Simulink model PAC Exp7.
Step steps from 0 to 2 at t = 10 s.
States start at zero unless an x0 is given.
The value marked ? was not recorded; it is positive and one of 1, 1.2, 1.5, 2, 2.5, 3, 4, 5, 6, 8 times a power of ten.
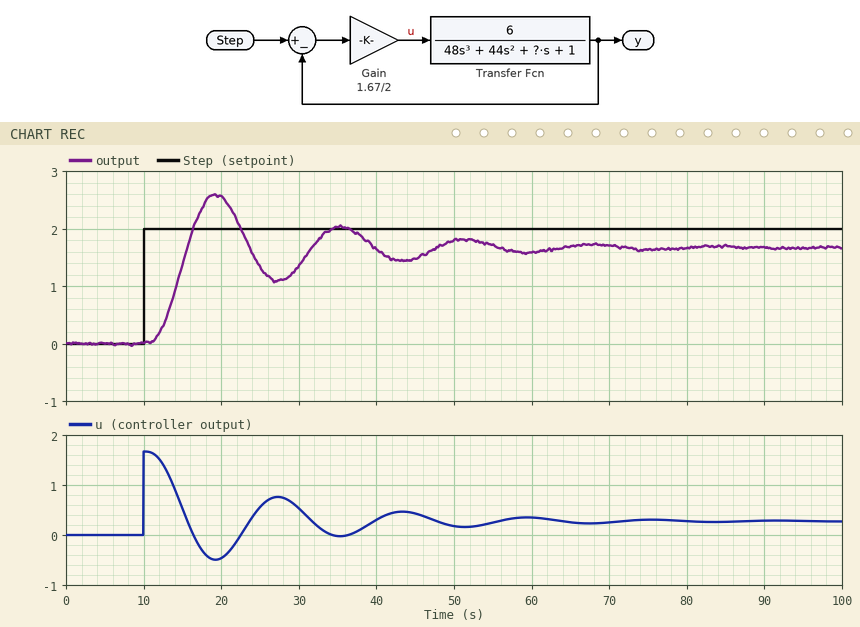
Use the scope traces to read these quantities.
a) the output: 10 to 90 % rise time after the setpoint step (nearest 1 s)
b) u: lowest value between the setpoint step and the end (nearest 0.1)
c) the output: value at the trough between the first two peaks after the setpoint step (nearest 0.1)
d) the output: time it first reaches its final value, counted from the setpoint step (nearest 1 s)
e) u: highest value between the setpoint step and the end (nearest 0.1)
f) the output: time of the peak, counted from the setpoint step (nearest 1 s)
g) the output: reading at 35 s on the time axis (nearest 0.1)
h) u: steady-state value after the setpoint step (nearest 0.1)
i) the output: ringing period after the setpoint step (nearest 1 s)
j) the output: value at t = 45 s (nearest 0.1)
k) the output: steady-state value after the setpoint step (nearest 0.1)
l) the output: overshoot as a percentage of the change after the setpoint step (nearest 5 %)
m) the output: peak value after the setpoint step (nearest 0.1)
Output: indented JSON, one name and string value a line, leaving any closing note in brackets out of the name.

{
  "the output: 10 to 90 % rise time after the setpoint step": "3 s",
  "u: lowest value between the setpoint step and the end": "-0.5",
  "the output: value at the trough between the first two peaks after the setpoint step": "1.1",
  "the output: time it first reaches its final value, counted from the setpoint step": "6 s",
  "u: highest value between the setpoint step and the end": "1.7",
  "the output: time of the peak, counted from the setpoint step": "9 s",
  "the output: reading at 35 s on the time axis": "2.0",
  "u: steady-state value after the setpoint step": "0.3",
  "the output: ringing period after the setpoint step": "16 s",
  "the output: value at t = 45 s": "1.5",
  "the output: steady-state value after the setpoint step": "1.7",
  "the output: overshoot as a percentage of the change after the setpoint step": "55 %",
  "the output: peak value after the setpoint step": "2.6"
}
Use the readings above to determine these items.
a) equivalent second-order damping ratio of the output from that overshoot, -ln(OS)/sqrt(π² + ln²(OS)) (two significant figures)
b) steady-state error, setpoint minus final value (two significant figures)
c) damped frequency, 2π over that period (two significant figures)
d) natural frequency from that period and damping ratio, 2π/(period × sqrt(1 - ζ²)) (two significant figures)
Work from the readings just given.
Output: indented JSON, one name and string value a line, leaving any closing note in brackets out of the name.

{
  "equivalent second-order damping ratio of the output from that overshoot, -ln(OS)/sqrt(π² + ln²(OS))": "0.19",
  "steady-state error, setpoint minus final value": "0.30",
  "damped frequency, 2π over that period": "0.39 rad/s",
  "natural frequency from that period and damping ratio, 2π/(period × sqrt(1 - ζ²))": "0.40 rad/s"
}
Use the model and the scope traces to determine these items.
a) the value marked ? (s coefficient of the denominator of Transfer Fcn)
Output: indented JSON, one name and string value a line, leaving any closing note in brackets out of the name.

{
  "the value marked ?": "12"
}
